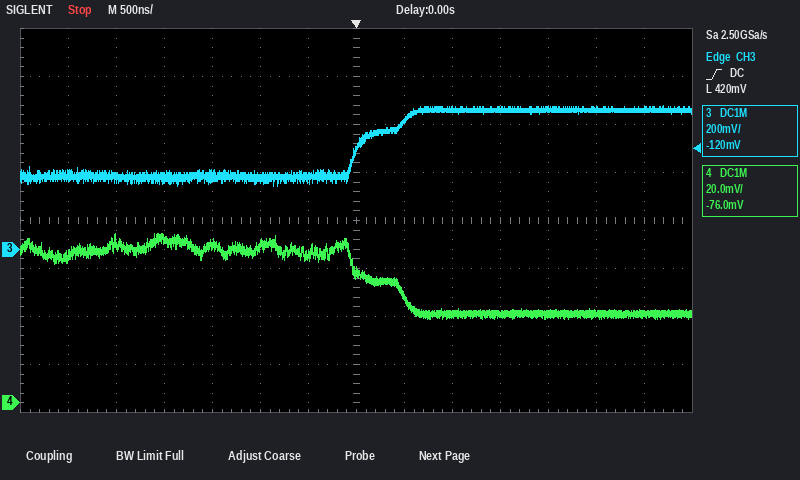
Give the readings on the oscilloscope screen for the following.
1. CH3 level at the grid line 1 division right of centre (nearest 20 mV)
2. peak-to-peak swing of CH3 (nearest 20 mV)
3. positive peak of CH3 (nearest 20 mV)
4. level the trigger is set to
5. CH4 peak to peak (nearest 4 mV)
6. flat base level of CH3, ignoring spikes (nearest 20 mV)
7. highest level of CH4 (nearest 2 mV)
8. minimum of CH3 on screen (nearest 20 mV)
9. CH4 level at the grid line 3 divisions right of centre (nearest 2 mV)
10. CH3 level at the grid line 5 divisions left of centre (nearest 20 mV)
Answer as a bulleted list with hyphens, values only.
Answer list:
- 540 mV
- 340 mV
- 600 mV
- 420 mV
- 36 mV
- 300 mV
- 70 mV
- 260 mV
- 38 mV
- 300 mV
